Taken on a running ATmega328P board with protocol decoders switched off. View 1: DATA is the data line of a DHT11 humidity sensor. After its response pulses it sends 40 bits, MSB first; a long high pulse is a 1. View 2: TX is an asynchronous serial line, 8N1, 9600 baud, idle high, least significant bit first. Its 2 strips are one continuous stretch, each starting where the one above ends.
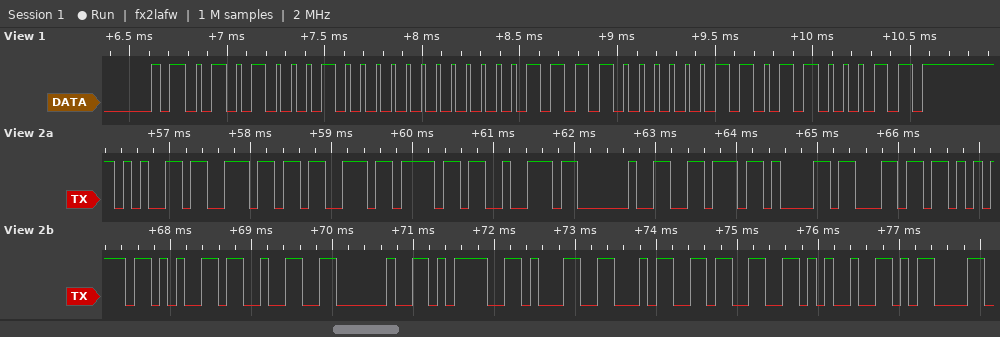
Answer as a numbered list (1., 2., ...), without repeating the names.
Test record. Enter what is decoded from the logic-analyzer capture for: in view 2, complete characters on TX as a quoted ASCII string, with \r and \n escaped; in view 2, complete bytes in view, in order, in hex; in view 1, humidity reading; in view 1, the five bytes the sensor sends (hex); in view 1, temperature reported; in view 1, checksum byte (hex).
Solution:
1. "ensor value2 =143%\r"
2. 65 6E 73 6F 72 20 76 61 6C 75 65 32 20 3D 31 34 33 25 0D
3. 81 %
4. 51 00 0F 03 63
5. 15.3 °C
6. 0x63
